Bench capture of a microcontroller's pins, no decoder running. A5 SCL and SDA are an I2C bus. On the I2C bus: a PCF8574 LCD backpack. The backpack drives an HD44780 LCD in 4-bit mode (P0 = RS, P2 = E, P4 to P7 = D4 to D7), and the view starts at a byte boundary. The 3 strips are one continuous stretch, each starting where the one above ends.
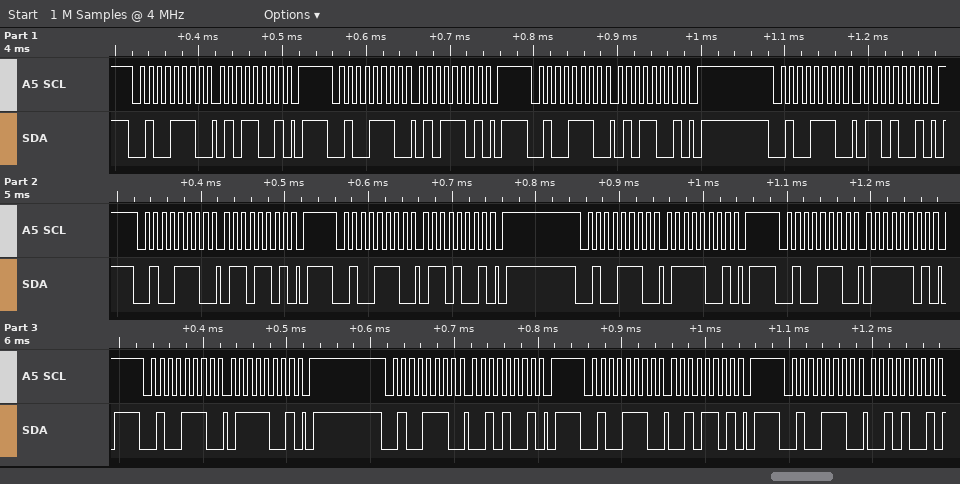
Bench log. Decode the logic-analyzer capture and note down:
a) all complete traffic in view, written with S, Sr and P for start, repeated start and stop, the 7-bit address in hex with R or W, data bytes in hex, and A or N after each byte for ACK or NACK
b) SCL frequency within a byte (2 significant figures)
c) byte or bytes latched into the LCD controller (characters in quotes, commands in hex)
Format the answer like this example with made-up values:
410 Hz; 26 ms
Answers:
S 27W A 59 A P S 27W A 5D A P S 27W A 59 A P S 27W A 69 A P S 27W A 6D A P S 27W A 69 A P S 27W A 79 A P S 27W A 7D A P S 27W A 79 A P S 27W A 29 A P S 27W A 2D A P S 27W A 29 A; 100 kHz; 'V' 'r'
